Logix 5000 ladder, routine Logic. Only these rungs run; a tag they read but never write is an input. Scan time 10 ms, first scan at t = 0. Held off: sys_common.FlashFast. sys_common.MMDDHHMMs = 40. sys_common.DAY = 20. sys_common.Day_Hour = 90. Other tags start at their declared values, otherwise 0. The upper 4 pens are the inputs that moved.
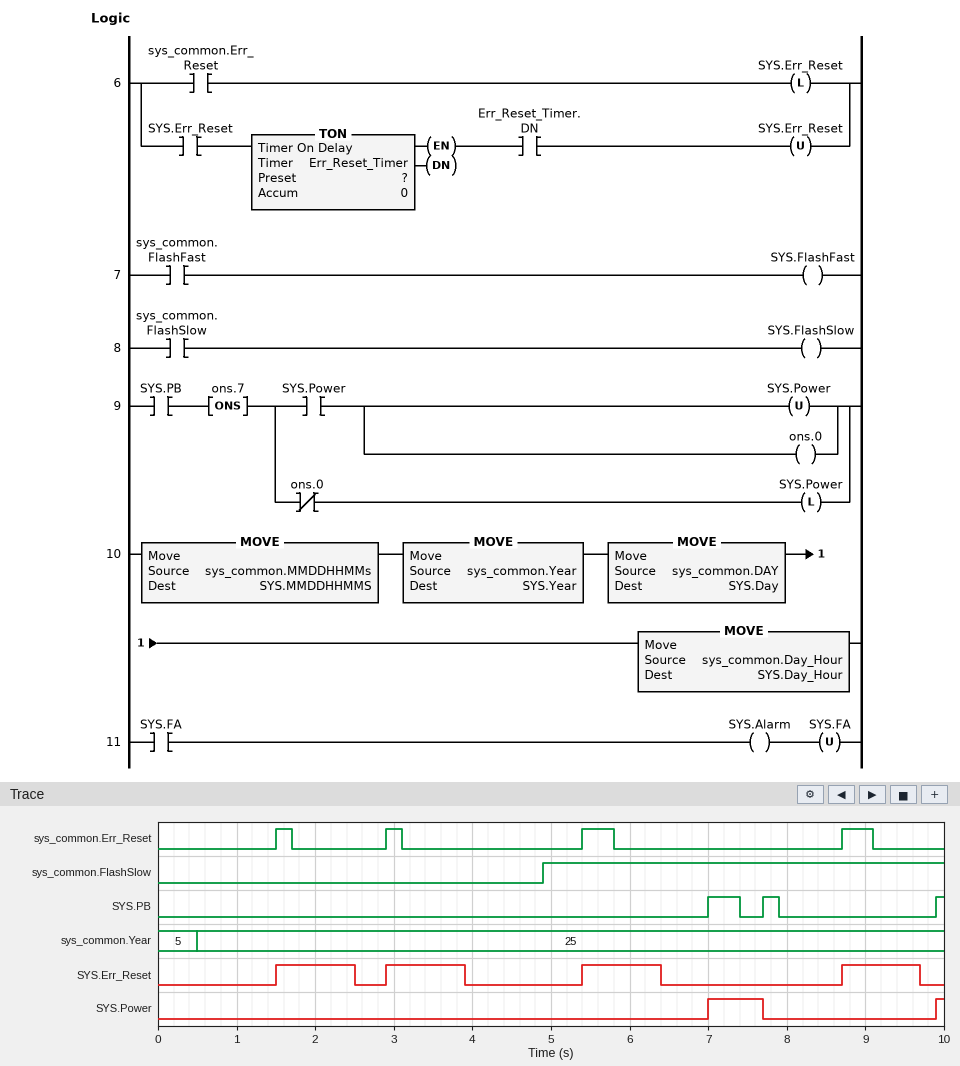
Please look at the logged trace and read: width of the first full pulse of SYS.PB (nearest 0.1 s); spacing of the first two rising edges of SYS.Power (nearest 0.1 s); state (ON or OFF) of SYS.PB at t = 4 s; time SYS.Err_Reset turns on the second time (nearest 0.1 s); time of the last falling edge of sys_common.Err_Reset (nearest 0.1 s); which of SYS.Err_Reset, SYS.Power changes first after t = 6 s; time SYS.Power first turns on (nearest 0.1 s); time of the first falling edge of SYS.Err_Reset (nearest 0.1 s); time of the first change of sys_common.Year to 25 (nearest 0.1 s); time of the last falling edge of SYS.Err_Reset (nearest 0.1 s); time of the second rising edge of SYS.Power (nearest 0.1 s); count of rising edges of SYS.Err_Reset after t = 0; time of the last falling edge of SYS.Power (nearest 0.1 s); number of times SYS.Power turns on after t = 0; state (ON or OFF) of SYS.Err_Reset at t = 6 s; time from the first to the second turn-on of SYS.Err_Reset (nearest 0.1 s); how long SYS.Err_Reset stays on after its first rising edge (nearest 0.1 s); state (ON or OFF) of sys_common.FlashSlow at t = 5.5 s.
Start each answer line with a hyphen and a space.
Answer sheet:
- 0.4 s
- 2.9 s
- OFF
- 2.9 s
- 9.1 s
- SYS.Err_Reset
- 7.0 s
- 2.5 s
- 0.5 s
- 9.7 s
- 9.9 s
- 4
- 7.7 s
- 2
- ON
- 1.4 s
- 1.0 s
- ON
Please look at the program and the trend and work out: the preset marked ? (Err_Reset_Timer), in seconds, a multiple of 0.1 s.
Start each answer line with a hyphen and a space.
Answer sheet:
- 1.0 s
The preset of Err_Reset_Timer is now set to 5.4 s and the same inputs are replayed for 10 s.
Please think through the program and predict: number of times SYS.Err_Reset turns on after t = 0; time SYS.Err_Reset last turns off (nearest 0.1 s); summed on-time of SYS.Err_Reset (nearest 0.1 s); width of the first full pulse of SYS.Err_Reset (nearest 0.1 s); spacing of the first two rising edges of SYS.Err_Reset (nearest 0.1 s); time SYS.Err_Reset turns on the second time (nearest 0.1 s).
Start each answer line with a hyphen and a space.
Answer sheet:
- 2
- 6.9 s
- 6.7 s
- 5.4 s
- 7.2 s
- 8.7 s
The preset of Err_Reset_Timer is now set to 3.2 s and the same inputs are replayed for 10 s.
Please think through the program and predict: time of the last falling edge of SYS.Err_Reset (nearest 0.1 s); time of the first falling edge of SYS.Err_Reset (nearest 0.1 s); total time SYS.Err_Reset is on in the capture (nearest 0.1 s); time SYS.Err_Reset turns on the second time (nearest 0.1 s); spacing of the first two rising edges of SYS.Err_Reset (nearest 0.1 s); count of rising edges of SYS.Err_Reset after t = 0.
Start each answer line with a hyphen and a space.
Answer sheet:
- 8.6 s
- 4.7 s
- 7.7 s
- 5.4 s
- 3.9 s
- 3
